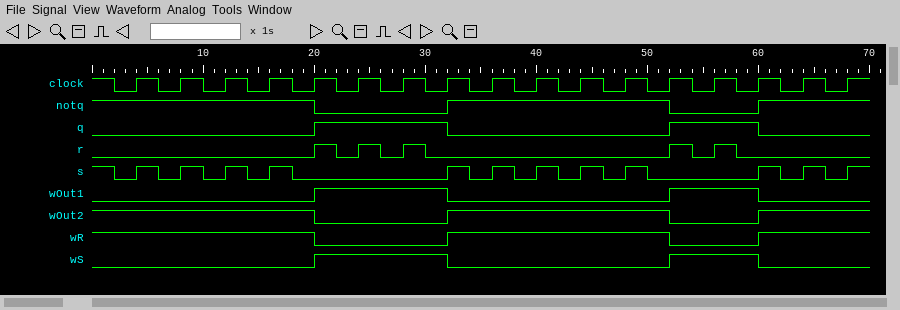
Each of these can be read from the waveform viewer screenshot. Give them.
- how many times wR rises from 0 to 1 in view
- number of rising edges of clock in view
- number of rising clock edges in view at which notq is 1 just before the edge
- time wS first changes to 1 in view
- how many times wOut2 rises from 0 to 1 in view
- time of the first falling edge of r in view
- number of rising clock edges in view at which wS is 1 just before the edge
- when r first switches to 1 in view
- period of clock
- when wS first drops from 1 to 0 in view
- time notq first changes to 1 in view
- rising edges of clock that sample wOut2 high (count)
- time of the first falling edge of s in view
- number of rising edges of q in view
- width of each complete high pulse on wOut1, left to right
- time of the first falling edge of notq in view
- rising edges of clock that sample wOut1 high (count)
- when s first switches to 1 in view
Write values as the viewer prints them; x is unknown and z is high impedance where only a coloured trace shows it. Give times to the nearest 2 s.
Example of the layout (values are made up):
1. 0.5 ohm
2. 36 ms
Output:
1. 2
2. 17
3. 12
4. 20 s
5. 2
6. 22 s
7. 5
8. 20 s
9. 4 s
10. 32 s
11. 32 s
12. 12
13. 2 s
14. 2
15. 12 s, 8 s
16. 20 s
17. 5
18. 4 s
